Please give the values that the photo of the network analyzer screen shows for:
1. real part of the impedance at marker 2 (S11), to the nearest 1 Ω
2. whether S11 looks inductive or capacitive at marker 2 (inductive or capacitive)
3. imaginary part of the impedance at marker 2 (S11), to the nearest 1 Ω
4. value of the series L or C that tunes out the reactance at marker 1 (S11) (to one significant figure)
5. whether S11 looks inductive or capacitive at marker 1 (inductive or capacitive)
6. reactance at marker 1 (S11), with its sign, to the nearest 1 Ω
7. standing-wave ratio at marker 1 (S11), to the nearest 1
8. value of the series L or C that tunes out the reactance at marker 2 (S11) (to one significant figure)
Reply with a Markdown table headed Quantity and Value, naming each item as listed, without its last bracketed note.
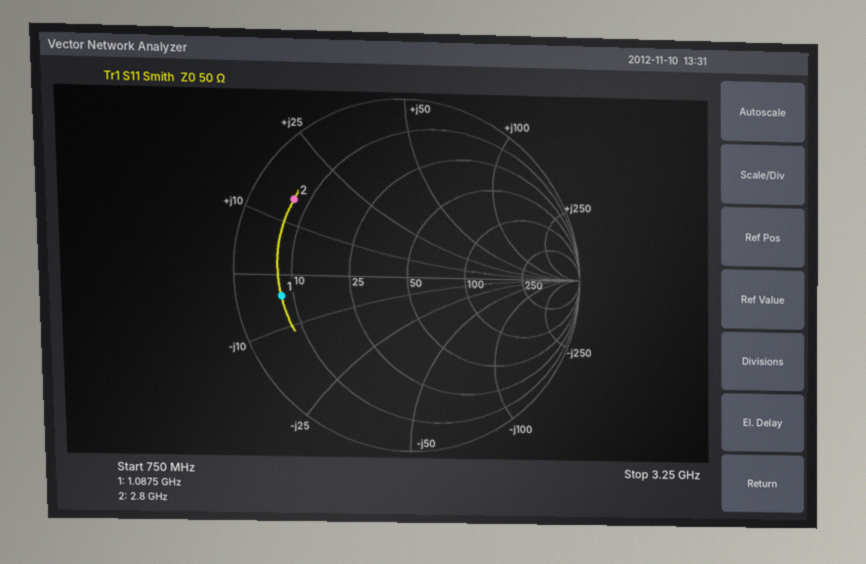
| Quantity | Value |
|---|---|
| real part of the impedance at marker 2 (S11), to the nearest 1 Ω | 7 Ω |
| whether S11 looks inductive or capacitive at marker 2 | inductive |
| imaginary part of the impedance at marker 2 (S11), to the nearest 1 Ω | +15 Ω |
| value of the series L or C that tunes out the reactance at marker 1 (S11) | 600 pH |
| whether S11 looks inductive or capacitive at marker 1 | capacitive |
| reactance at marker 1 (S11), with its sign, to the nearest 1 Ω | -4 Ω |
| standing-wave ratio at marker 1 (S11), to the nearest 1 | 7 |
| value of the series L or C that tunes out the reactance at marker 2 (S11) | 4 pF |
